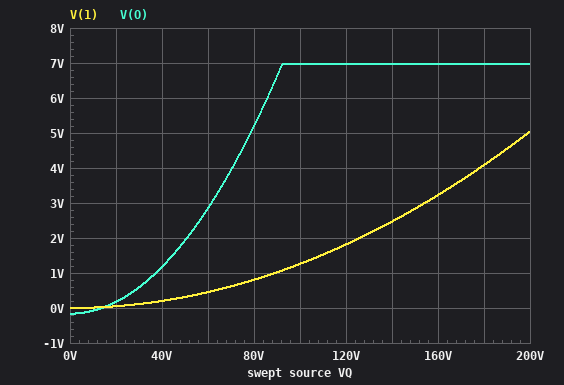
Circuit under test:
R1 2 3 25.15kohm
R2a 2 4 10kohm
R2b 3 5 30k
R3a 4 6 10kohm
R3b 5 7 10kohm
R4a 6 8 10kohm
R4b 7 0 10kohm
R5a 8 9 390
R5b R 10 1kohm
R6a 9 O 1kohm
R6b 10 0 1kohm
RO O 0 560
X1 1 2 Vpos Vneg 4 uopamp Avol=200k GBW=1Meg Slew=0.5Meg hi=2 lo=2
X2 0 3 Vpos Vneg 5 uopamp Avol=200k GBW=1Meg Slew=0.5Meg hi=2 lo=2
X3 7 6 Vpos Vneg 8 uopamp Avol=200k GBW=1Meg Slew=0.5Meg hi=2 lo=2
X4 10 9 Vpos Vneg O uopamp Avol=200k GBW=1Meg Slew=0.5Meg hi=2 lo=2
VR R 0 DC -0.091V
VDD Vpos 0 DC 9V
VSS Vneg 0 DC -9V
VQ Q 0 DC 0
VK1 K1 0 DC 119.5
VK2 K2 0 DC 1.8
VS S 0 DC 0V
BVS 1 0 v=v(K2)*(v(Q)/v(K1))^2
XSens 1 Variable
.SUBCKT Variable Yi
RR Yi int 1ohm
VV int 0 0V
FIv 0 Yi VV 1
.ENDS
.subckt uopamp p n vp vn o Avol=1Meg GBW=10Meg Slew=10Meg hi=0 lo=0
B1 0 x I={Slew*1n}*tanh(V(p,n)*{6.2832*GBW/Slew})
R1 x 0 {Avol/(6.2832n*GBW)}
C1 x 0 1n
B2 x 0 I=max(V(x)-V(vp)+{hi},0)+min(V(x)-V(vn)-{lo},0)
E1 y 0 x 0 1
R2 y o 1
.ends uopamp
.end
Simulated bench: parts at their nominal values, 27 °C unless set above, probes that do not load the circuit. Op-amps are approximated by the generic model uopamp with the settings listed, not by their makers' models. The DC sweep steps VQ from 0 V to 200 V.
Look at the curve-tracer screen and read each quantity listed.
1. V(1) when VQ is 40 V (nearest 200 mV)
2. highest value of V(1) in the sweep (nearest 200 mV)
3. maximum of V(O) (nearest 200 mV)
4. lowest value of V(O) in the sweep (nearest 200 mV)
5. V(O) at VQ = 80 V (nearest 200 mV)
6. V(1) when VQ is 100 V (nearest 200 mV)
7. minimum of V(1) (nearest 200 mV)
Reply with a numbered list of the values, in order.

1. 200 mV
2. 5.0 V
3. 7.0 V
4. -200 mV
5. 5.2 V
6. 1.2 V
7. 0 V
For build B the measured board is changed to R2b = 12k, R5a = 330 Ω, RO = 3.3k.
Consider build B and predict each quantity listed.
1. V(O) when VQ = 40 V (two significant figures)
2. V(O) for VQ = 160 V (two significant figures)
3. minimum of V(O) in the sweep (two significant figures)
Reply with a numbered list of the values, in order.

1. 960 mV
2. 7.0 V
3. -180 mV
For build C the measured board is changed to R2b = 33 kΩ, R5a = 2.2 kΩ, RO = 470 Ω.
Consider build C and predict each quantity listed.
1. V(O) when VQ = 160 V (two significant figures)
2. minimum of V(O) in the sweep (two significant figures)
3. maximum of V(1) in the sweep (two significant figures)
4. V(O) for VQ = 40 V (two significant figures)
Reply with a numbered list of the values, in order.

1. 3.1 V
2. -66 mV
3. 5.0 V
4. 180 mV
